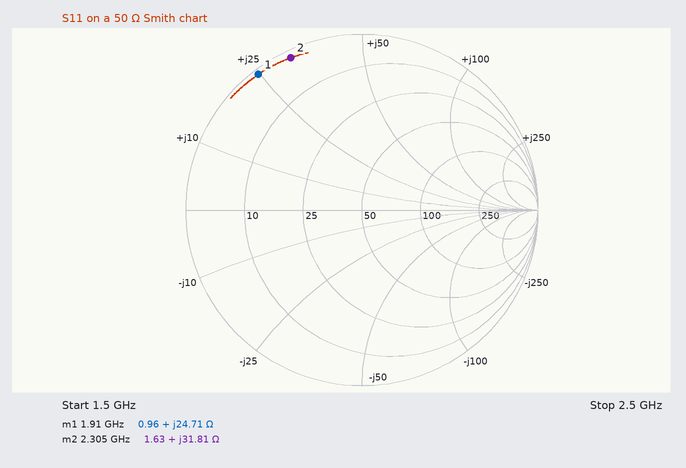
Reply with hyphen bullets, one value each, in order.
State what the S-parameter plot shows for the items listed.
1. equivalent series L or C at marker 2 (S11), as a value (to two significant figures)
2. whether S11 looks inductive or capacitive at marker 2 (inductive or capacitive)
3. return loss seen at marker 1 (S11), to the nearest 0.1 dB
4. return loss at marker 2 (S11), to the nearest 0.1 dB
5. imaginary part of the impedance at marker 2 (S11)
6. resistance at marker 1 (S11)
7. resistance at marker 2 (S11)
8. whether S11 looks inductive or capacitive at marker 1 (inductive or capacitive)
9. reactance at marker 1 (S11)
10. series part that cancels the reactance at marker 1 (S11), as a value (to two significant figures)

- 2.2 nH
- inductive
- 0.3 dB
- 0.4 dB
- +31.81 Ω
- 0.96 Ω
- 1.63 Ω
- inductive
- +24.71 Ω
- 3.4 pF
